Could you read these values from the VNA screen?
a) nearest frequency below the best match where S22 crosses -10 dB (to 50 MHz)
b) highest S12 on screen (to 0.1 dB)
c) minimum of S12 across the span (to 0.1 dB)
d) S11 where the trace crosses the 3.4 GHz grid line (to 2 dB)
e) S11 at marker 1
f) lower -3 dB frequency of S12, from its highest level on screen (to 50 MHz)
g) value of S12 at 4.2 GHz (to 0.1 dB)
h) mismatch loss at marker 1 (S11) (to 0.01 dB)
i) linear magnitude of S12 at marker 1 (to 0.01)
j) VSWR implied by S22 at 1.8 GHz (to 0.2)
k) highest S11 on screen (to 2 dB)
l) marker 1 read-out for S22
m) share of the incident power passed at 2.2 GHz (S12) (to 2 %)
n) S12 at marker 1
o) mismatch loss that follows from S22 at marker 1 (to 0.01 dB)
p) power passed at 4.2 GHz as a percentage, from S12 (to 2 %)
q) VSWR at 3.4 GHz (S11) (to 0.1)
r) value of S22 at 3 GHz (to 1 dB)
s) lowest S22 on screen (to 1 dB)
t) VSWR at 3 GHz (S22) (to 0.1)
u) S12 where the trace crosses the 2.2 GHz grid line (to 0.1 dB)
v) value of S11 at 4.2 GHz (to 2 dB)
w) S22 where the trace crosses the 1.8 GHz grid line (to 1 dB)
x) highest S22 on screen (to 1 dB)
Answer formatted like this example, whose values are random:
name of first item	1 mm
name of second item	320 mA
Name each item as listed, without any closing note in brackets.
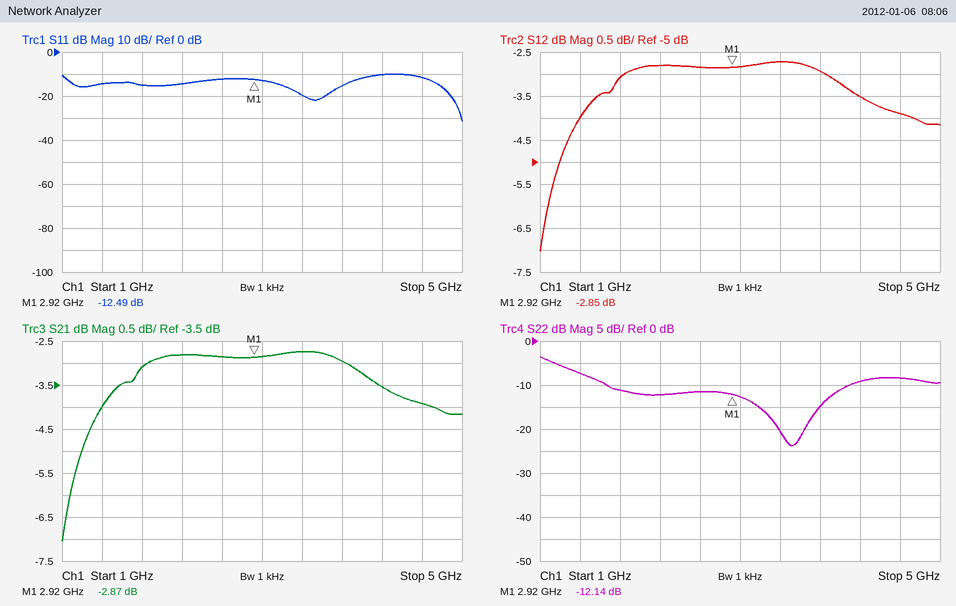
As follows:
nearest frequency below the best match where S22 crosses -10 dB	1.65 GHz
highest S12 on screen	-2.7 dB
minimum of S12 across the span	-7.0 dB
S11 where the trace crosses the 3.4 GHz grid line	-20 dB
S11 at marker 1	-12.49 dB
lower -3 dB frequency of S12, from its highest level on screen	1.10 GHz
value of S12 at 4.2 GHz	-3.5 dB
mismatch loss at marker 1 (S11)	0.25 dB
linear magnitude of S12 at marker 1	0.72
VSWR implied by S22 at 1.8 GHz	1.8
highest S11 on screen	-10 dB
marker 1 read-out for S22	-12.14 dB
share of the incident power passed at 2.2 GHz (S12)	52 %
S12 at marker 1	-2.85 dB
mismatch loss that follows from S22 at marker 1	0.27 dB
power passed at 4.2 GHz as a percentage, from S12	44 %
VSWR at 3.4 GHz (S11)	1.2
value of S22 at 3 GHz	-13 dB
lowest S22 on screen	-24 dB
VSWR at 3 GHz (S22)	1.6
S12 where the trace crosses the 2.2 GHz grid line	-2.8 dB
value of S11 at 4.2 GHz	-10 dB
S22 where the trace crosses the 1.8 GHz grid line	-11 dB
highest S22 on screen	-4 dB
